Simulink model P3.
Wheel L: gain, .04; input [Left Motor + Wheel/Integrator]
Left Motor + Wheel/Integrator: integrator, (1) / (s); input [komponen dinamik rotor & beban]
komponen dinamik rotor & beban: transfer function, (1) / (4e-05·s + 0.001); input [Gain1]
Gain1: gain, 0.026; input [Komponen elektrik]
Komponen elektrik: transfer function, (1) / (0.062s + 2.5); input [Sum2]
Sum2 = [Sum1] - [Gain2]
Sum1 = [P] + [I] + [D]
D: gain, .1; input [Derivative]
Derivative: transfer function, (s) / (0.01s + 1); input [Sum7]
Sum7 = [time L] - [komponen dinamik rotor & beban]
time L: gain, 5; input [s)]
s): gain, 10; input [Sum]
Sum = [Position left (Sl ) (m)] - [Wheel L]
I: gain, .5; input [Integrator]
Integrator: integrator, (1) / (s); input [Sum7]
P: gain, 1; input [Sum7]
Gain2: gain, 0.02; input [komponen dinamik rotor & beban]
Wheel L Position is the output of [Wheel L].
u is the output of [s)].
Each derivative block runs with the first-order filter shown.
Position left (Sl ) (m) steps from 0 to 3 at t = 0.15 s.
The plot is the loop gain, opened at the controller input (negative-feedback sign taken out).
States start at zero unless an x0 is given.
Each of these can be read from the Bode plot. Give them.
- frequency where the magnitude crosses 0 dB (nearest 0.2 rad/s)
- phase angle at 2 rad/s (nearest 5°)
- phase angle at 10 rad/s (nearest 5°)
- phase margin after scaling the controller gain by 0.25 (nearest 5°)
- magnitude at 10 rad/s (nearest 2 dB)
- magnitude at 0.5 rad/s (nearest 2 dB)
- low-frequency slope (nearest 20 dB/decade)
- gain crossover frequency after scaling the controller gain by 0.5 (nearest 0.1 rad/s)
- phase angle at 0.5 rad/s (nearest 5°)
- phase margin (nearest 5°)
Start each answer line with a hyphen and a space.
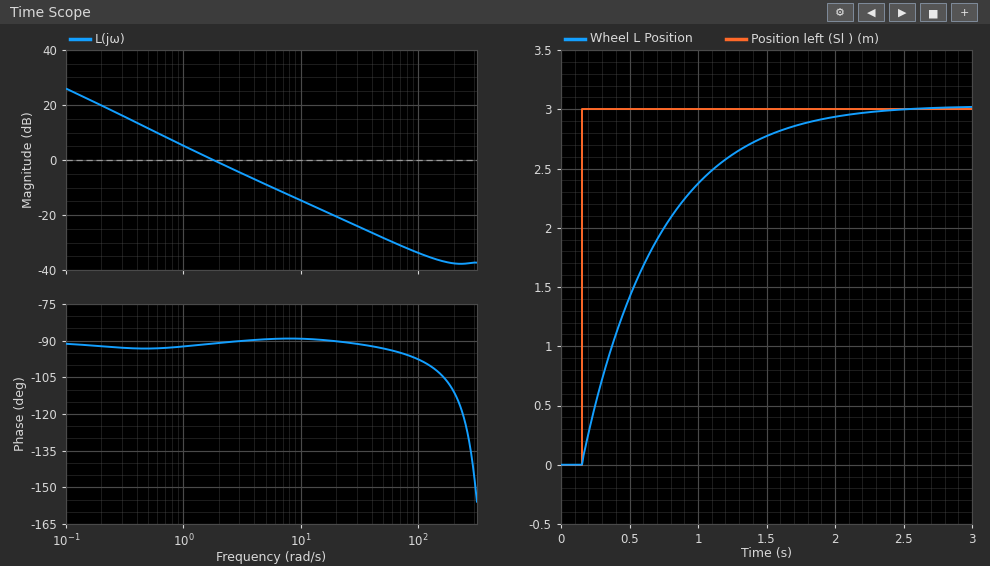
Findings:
- 1.8 rad/s
- -90°
- -90°
- 85°
- -14 dB
- 12 dB
- -20 dB/decade
- 0.9 rad/s
- -95°
- 90°
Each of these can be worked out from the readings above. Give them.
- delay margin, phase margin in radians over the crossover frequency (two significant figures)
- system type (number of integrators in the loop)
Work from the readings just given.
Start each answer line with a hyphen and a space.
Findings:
- 0.87 s
- 1
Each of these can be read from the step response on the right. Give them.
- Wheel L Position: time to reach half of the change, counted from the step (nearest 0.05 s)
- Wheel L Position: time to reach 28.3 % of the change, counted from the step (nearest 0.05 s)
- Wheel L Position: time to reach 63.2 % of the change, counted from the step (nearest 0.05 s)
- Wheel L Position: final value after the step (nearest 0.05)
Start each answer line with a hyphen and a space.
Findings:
- 0.40 s
- 0.20 s
- 0.55 s
- 3.00
